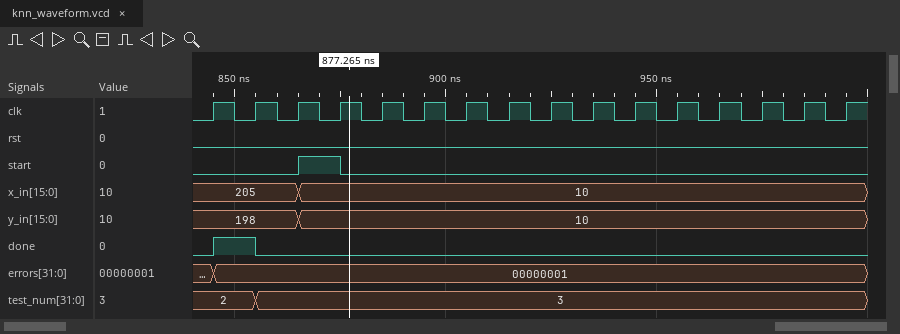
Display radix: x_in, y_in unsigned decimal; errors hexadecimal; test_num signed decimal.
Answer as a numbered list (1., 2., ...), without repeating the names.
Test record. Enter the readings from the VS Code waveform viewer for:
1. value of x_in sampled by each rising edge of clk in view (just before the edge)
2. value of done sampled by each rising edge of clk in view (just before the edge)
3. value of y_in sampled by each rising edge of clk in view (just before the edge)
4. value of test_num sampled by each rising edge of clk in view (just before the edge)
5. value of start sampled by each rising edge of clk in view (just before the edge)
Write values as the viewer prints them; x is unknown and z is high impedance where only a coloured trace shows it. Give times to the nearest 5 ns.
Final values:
1. 205, 205, 205, 10, 10, 10, 10, 10, 10, 10, 10, 10, 10, 10, 10, 10
2. 0 1 0 0 0 0 0 0 0 0 0 0 0 0 0 0
3. 198, 198, 198, 10, 10, 10, 10, 10, 10, 10, 10, 10, 10, 10, 10, 10
4. 2, 2, 3, 3, 3, 3, 3, 3, 3, 3, 3, 3, 3, 3, 3, 3
5. 0 0 0 1 0 0 0 0 0 0 0 0 0 0 0 0
